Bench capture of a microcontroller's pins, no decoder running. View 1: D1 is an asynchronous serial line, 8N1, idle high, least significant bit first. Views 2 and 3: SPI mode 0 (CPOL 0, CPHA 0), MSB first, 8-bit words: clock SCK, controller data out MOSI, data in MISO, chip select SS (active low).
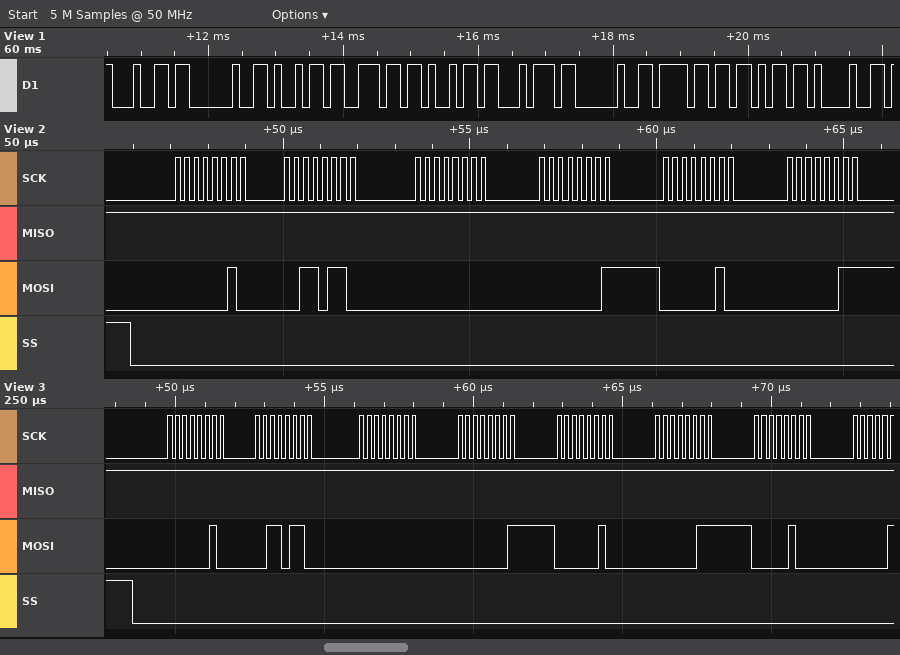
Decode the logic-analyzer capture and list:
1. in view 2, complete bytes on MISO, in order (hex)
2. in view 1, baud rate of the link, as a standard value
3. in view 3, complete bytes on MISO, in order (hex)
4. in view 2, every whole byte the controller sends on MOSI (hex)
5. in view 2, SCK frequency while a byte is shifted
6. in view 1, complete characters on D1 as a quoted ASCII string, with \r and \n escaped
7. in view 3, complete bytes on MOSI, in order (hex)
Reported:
FF FF FF FF FF FF
9600 baud
0xFF 0xFF 0xFF 0xFF 0xFF 0xFF 0xFF
02 36 00 01 02 03
4 MHz
"d init ok!"
0x02 0x36 0x00 0x01 0x02 0x03 0x04
